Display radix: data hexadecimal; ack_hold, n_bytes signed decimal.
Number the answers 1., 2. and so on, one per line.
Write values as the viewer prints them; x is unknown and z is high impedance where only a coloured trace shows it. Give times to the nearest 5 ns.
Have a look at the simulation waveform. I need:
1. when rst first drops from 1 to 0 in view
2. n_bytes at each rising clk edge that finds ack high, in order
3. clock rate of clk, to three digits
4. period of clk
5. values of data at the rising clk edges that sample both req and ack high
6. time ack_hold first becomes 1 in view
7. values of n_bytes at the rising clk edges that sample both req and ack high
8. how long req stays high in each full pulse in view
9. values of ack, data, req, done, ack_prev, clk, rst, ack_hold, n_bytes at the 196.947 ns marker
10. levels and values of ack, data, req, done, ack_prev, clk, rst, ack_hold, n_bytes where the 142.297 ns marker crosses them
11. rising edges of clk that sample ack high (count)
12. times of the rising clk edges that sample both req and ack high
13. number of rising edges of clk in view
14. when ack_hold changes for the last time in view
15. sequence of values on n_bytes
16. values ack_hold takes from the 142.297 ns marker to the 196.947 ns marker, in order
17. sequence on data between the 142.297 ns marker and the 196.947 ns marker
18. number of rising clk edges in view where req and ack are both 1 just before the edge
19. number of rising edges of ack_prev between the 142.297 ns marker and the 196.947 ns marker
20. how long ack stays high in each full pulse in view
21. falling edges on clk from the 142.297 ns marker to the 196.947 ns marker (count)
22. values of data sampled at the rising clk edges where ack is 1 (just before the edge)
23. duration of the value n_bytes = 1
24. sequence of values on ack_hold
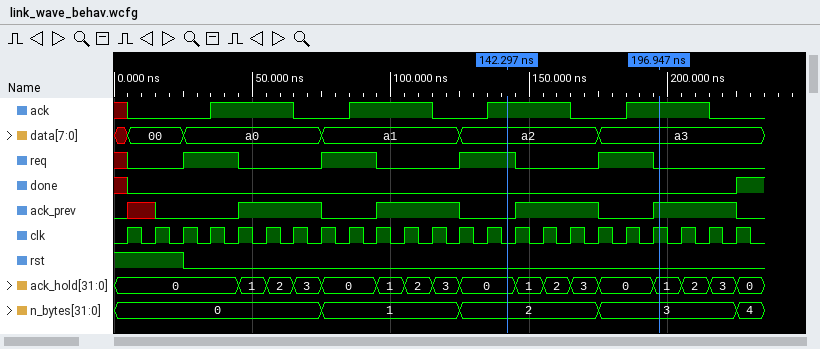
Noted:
1. 25 ns
2. 0, 0, 0, 1, 1, 1, 2, 2, 2, 3, 3, 3
3. 100 MHz
4. 10 ns
5. a0, a1, a2, a3
6. 45 ns
7. 0, 1, 2, 3
8. 20 ns, 20 ns, 20 ns, 20 ns
9. ack=1, data=a3, req=0, done=0, ack_prev=1, clk=1, rst=0, ack_hold=1, n_bytes=3
10. ack=1, data=a2, req=1, done=0, ack_prev=0, clk=0, rst=0, ack_hold=0, n_bytes=2
11. 12
12. 45 ns, 95 ns, 145 ns, 195 ns
13. 23
14. 225 ns
15. 0, 1, 2, 3, 4
16. 0, 1, 2, 3, 0, 1
17. a2, a3
18. 4
19. 2
20. 30 ns, 30 ns, 30 ns, 30 ns
21. 5
22. a0, a0, a0, a1, a1, a1, a2, a2, a2, a3, a3, a3
23. 50 ns
24. 0, 1, 2, 3, 0, 1, 2, 3, 0, 1, 2, 3, 0, 1, 2, 3, 0
